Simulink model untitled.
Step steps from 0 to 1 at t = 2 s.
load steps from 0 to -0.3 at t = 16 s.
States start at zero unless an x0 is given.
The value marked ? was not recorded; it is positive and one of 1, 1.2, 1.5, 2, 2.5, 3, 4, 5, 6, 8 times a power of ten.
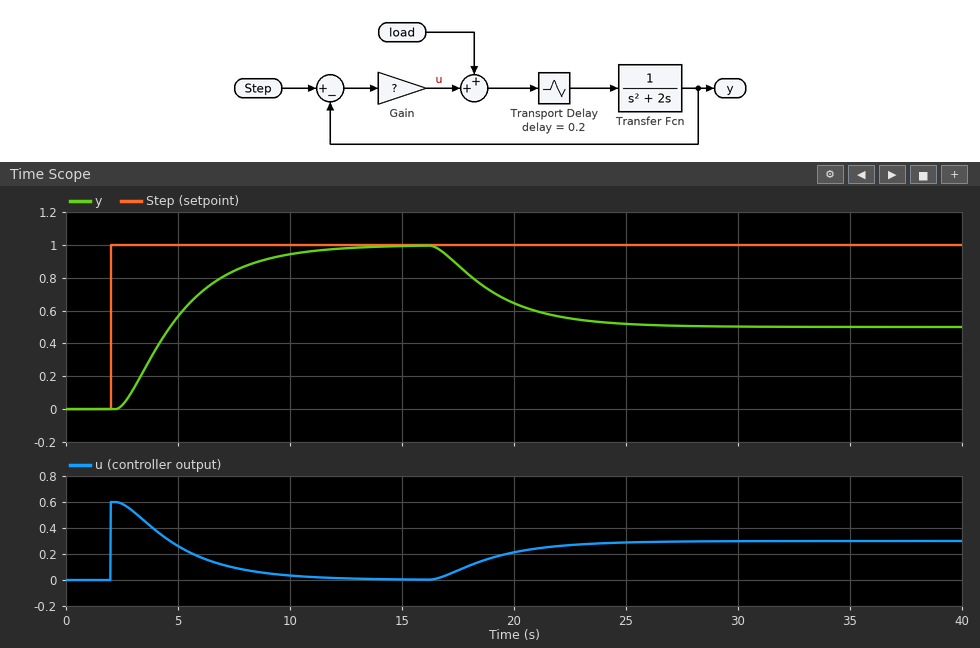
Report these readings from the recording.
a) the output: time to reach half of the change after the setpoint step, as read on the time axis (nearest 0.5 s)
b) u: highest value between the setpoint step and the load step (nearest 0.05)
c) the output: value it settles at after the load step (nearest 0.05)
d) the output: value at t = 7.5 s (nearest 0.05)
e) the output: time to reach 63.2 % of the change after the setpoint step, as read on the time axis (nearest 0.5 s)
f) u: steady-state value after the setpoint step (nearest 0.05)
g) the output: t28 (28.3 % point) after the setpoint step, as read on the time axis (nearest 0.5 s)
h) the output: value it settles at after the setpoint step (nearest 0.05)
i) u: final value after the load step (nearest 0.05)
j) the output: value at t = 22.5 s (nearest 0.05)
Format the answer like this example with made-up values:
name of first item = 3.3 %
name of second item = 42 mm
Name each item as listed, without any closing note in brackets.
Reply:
the output: time to reach half of the change after the setpoint step, as read on the time axis = 4.5 s
u: highest value between the setpoint step and the load step = 0.60
the output: value it settles at after the load step = 0.50
the output: value at t = 7.5 s = 0.85
the output: time to reach 63.2 % of the change after the setpoint step, as read on the time axis = 5.5 s
u: steady-state value after the setpoint step = 0.00
the output: t28 (28.3 % point) after the setpoint step, as read on the time axis = 3.5 s
the output: value it settles at after the setpoint step = 1.00
u: final value after the load step = 0.30
the output: value at t = 22.5 s = 0.55
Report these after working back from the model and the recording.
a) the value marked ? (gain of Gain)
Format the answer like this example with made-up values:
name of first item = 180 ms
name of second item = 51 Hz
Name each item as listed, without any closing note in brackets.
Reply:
the value marked ? = 0.6
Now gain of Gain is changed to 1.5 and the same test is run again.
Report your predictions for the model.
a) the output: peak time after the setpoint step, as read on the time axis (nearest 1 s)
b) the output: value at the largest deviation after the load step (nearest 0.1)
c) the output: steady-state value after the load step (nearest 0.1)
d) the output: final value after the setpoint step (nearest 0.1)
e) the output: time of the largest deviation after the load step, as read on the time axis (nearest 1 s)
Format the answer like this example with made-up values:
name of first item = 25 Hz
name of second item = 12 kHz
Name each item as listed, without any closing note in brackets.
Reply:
the output: peak time after the setpoint step, as read on the time axis = 6 s
the output: value at the largest deviation after the load step = 0.8
the output: steady-state value after the load step = 0.8
the output: final value after the setpoint step = 1.0
the output: time of the largest deviation after the load step, as read on the time axis = 20 s
